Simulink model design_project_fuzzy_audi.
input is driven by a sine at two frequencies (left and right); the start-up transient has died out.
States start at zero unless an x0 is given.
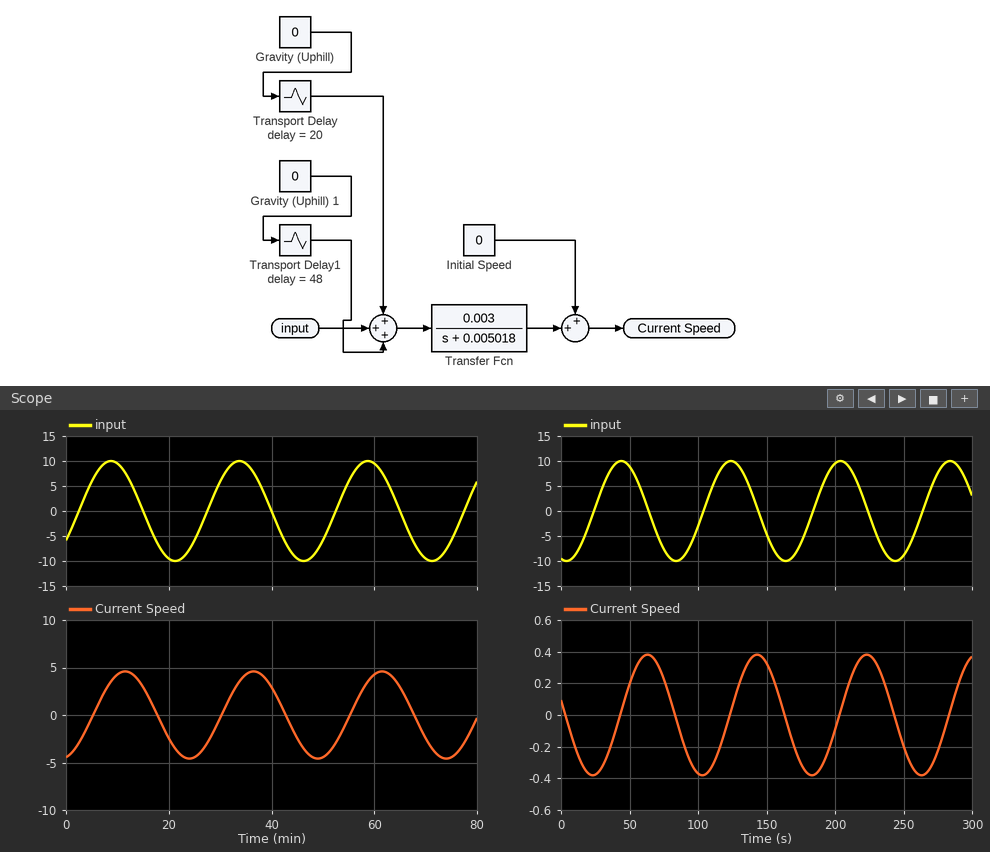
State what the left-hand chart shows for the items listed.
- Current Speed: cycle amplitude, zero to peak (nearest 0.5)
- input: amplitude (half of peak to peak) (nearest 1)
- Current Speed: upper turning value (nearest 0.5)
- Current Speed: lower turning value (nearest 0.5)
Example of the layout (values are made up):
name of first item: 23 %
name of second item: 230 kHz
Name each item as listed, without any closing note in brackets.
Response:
Current Speed: cycle amplitude, zero to peak: 4.5
input: amplitude (half of peak to peak): 10
Current Speed: upper turning value: 4.5
Current Speed: lower turning value: -4.5
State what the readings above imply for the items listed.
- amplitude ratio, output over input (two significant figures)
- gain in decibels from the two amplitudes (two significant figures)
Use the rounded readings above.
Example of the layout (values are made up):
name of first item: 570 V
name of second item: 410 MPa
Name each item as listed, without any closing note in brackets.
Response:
amplitude ratio, output over input: 0.45
gain in decibels from the two amplitudes: -6.9 dB
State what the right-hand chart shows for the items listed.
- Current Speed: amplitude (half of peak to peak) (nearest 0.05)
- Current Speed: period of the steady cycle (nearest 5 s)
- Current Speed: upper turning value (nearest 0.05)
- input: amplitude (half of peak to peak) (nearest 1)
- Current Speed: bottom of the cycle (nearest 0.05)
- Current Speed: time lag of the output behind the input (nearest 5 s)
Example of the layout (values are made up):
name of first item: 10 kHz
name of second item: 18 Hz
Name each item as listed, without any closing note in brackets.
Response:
Current Speed: amplitude (half of peak to peak): 0.40
Current Speed: period of the steady cycle: 80 s
Current Speed: upper turning value: 0.40
input: amplitude (half of peak to peak): 10
Current Speed: bottom of the cycle: -0.40
Current Speed: time lag of the output behind the input: 20 s
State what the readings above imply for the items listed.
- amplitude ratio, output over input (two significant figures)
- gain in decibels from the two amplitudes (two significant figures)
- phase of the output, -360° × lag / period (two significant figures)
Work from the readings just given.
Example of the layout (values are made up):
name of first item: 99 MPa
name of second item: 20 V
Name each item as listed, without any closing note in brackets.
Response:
amplitude ratio, output over input: 0.040
gain in decibels from the two amplitudes: -28 dB
phase of the output, -360° × lag / period: -90°
